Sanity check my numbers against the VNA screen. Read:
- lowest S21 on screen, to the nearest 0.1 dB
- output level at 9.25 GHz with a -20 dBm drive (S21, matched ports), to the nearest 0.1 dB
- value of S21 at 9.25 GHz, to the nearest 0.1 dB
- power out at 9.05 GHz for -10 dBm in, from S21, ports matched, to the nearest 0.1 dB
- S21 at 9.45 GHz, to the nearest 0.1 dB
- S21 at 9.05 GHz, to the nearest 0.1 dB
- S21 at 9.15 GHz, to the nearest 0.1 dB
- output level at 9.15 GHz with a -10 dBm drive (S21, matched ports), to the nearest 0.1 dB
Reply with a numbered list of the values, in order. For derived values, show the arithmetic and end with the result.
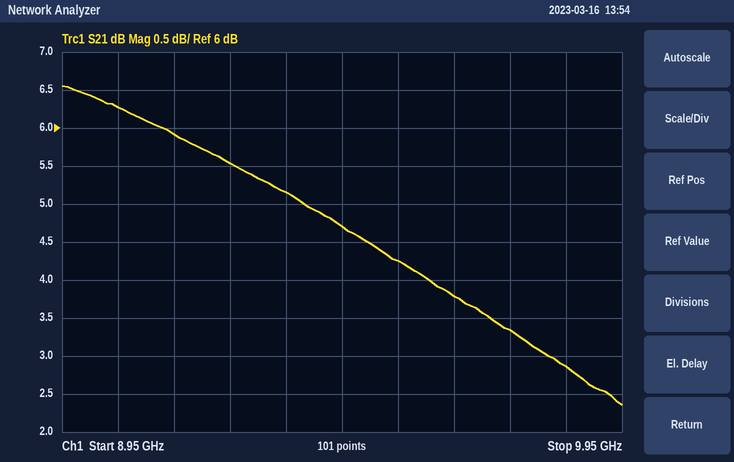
1. 2.4 dB
2. -20 dBm + (5.5 dB) = -14.5 dBm
3. 5.5 dB
4. -10 dBm + (6.3 dB) = -3.7 dBm
5. 4.7 dB
6. 6.3 dB
7. 5.9 dB
8. -10 dBm + (5.9 dB) = -4.1 dBm
